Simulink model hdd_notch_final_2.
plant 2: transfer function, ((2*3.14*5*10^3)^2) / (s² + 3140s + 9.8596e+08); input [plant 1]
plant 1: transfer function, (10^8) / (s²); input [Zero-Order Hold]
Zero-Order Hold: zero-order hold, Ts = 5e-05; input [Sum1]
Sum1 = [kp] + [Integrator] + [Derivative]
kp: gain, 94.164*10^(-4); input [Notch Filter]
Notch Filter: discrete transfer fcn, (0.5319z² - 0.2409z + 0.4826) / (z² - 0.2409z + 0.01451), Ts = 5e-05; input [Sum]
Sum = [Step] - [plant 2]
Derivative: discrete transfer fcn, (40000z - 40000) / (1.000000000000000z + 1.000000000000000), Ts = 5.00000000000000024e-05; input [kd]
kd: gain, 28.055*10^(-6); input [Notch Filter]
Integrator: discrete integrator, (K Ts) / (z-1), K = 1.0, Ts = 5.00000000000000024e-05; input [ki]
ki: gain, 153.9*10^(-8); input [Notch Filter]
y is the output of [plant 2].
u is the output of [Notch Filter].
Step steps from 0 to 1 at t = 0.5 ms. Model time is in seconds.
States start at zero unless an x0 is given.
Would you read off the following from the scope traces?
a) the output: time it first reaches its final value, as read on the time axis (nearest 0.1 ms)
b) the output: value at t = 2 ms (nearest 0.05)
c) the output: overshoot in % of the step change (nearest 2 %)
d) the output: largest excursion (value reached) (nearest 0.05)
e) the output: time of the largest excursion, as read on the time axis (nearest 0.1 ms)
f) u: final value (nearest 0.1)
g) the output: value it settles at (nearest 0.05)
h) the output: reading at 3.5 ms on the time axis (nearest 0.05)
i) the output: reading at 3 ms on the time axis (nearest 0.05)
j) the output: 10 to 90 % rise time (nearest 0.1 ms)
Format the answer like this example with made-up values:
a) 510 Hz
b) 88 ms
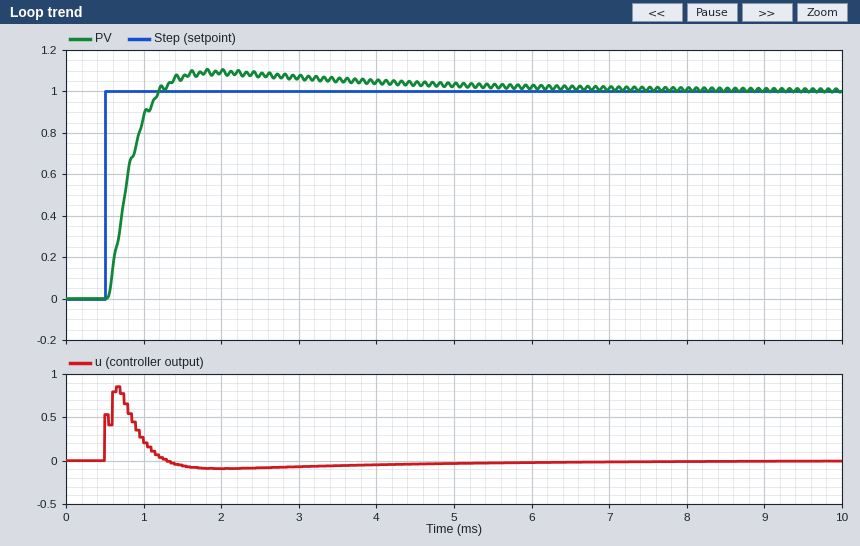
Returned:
a) 1.2 ms
b) 1.10
c) 10 %
d) 1.10
e) 1.8 ms
f) 0.0
g) 1.00
h) 1.05
i) 1.05
j) 0.4 ms
